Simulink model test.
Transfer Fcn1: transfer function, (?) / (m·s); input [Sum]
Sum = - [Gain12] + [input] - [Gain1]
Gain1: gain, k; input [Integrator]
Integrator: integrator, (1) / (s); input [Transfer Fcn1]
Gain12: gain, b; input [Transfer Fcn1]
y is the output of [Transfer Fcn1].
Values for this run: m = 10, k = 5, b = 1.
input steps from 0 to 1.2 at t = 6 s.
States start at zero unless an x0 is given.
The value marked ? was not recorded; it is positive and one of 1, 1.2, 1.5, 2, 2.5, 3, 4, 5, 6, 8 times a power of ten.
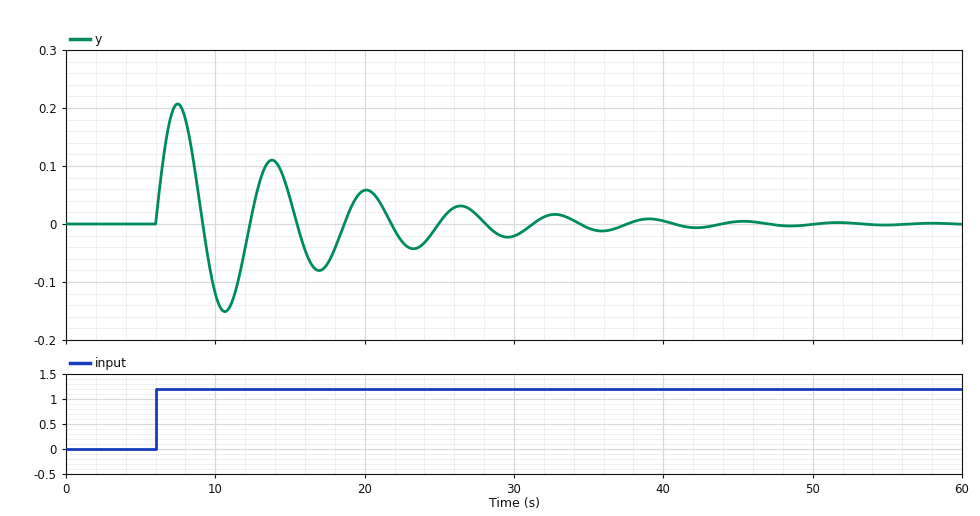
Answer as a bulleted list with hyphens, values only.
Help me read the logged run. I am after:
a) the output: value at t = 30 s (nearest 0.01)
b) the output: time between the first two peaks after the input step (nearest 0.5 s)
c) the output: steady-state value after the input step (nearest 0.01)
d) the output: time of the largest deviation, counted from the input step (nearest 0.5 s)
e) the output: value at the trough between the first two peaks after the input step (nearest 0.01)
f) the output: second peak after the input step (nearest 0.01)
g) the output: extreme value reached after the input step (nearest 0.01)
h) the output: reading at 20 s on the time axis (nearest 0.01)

- -0.02
- 6.5 s
- 0.00
- 1.5 s
- -0.15
- 0.11
- 0.21
- 0.06
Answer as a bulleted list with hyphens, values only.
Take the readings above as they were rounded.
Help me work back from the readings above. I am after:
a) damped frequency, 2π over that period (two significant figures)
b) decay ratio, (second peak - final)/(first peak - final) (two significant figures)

- 0.97 rad/s
- 0.52
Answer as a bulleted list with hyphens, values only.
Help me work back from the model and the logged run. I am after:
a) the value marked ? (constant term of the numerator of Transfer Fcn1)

- 2
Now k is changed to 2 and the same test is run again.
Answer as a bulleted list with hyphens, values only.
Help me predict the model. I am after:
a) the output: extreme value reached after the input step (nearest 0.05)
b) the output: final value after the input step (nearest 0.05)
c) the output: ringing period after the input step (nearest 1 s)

- 0.30
- 0.00
- 10 s
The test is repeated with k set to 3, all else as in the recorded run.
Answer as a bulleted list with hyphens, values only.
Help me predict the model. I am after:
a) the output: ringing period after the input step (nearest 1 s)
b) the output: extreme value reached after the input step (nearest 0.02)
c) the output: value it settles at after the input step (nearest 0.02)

- 8 s
- 0.26
- 0.00
